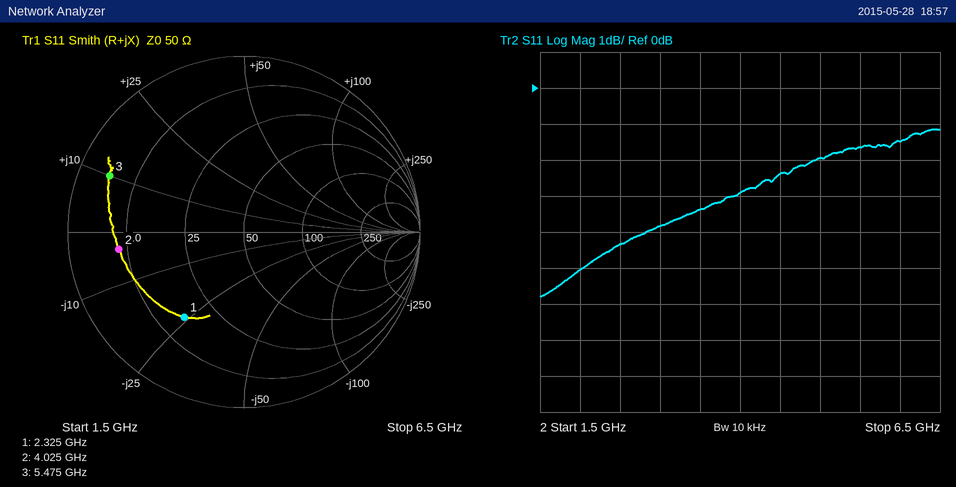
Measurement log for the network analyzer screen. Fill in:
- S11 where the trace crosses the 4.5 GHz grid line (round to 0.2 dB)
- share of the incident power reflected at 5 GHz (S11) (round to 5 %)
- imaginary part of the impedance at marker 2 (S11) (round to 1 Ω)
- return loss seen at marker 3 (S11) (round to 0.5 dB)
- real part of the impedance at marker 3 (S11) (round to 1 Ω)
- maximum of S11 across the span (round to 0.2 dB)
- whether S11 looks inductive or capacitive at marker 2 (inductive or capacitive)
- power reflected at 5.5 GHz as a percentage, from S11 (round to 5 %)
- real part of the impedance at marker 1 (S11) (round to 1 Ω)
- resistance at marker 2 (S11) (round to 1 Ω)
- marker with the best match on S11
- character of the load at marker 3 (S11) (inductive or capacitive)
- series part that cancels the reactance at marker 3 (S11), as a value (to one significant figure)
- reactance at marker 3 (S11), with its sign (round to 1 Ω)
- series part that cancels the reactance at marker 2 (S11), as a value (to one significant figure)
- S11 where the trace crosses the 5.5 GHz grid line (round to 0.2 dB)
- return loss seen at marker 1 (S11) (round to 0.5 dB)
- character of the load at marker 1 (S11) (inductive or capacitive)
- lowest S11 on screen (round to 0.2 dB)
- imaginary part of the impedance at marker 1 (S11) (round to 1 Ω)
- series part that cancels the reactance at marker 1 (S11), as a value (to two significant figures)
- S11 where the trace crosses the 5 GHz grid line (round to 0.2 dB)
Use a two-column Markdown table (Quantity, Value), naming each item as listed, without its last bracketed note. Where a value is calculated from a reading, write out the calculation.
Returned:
| Quantity | Value |
|---|---|
| S11 where the trace crosses the 4.5 GHz grid line | -2.4 dB |
| share of the incident power reflected at 5 GHz (S11) | 10^(-2/10) ≈ 63.1 %, so 65 % to the nearest 5 % |
| imaginary part of the impedance at marker 2 (S11) | -3 Ω |
| return loss seen at marker 3 (S11) | 1.5 dB |
| real part of the impedance at marker 3 (S11) | 5 Ω |
| maximum of S11 across the span | -1.2 dB |
| whether S11 looks inductive or capacitive at marker 2 | capacitive |
| power reflected at 5.5 GHz as a percentage, from S11 | 10^(-1.6/10) ≈ 69.2 %, so 70 % to the nearest 5 % |
| real part of the impedance at marker 1 (S11) | 16 Ω |
| resistance at marker 2 (S11) | 8 Ω |
| marker with the best match on S11 | marker 1 |
| character of the load at marker 3 (S11) | inductive |
| series part that cancels the reactance at marker 3 (S11), as a value | C = 1/(2π × 5.475 GHz × 10 Ω) ≈ 3 pF |
| reactance at marker 3 (S11), with its sign | +10 Ω |
| series part that cancels the reactance at marker 2 (S11), as a value | L = 3 Ω/(2π × 4.025 GHz) ≈ 119 pH, so 100 pH to one significant figure |
| S11 where the trace crosses the 5.5 GHz grid line | -1.6 dB |
| return loss seen at marker 1 (S11) | 4.5 dB |
| character of the load at marker 1 (S11) | capacitive |
| lowest S11 on screen | -5.8 dB |
| imaginary part of the impedance at marker 1 (S11) | -24 Ω |
| series part that cancels the reactance at marker 1 (S11), as a value | L = 24 Ω/(2π × 2.325 GHz) ≈ 1.6 nH |
| S11 where the trace crosses the 5 GHz grid line | -2.0 dB |
